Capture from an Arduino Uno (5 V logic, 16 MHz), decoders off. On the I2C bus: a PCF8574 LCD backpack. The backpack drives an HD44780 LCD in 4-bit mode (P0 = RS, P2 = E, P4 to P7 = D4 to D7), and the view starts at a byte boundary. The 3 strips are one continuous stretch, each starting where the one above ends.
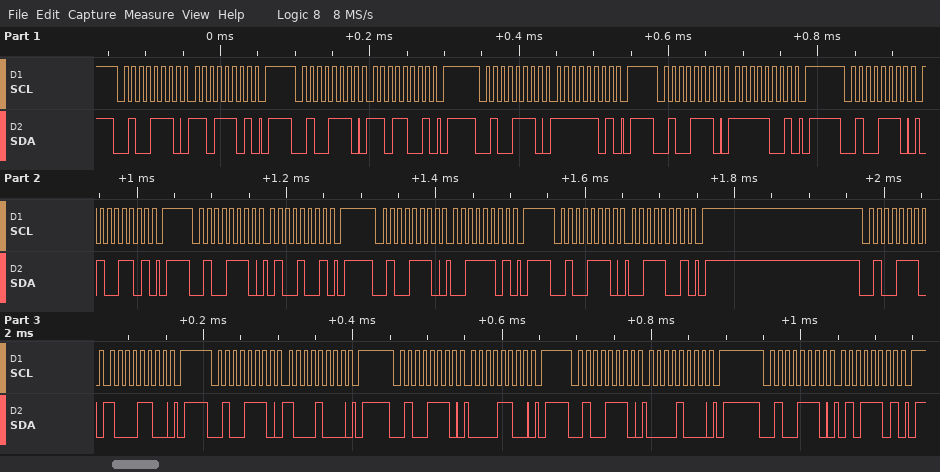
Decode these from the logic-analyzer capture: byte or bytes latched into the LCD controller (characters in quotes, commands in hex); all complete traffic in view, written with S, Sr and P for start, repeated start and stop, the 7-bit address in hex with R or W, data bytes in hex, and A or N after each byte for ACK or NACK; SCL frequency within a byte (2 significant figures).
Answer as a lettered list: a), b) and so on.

a) data 0xDF 'C' 0x80
b) S 27W A DD A P S 27W A D9 A P S 27W A FD A P S 27W A F9 A P S 27W A 4D A P S 27W A 49 A P S 27W A 3D A P S 27W A 39 A P S 27W A 8C A P S 27W A 88 A P S 27W A 0C A P S 27W A 08 A P S 27W A 5D A P
c) 100 kHz
